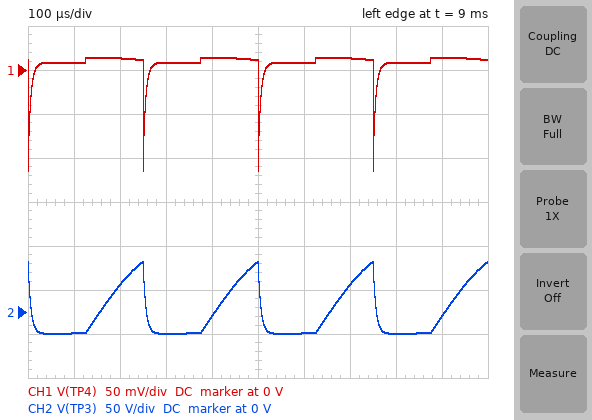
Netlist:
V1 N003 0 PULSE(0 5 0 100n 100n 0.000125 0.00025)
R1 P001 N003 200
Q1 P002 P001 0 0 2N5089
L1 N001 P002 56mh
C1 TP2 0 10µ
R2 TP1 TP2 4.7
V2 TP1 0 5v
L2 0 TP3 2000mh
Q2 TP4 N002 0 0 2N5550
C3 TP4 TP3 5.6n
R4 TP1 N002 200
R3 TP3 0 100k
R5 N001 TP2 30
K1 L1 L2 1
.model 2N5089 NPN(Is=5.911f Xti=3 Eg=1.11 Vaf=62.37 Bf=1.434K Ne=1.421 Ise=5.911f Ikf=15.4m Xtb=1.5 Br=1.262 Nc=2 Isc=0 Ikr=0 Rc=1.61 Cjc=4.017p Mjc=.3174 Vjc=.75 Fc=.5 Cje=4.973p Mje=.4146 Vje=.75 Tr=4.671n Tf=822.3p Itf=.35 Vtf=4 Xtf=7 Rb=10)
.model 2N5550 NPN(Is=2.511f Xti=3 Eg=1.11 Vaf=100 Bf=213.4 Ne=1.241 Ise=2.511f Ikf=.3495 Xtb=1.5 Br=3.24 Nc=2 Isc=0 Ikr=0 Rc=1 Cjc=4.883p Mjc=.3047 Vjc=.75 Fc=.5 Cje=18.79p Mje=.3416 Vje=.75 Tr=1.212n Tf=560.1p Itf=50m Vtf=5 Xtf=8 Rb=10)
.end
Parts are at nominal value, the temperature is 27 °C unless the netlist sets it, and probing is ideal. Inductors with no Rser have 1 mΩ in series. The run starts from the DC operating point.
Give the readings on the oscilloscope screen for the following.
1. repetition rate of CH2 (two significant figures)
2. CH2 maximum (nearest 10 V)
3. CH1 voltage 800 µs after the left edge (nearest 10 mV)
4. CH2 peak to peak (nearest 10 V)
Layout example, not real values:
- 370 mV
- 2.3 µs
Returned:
- 4.0 kHz
- 60 V
- 10 mV
- 80 V
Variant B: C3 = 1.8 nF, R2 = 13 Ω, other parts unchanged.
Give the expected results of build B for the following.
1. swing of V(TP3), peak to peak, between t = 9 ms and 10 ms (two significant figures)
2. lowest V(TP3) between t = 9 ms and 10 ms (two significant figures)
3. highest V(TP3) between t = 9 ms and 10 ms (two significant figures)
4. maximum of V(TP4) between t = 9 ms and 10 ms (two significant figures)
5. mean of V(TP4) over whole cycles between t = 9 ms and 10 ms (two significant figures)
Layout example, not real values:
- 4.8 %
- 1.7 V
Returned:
- 79 V
- -28 V
- 51 V
- 11 mV
- 8.2 mV
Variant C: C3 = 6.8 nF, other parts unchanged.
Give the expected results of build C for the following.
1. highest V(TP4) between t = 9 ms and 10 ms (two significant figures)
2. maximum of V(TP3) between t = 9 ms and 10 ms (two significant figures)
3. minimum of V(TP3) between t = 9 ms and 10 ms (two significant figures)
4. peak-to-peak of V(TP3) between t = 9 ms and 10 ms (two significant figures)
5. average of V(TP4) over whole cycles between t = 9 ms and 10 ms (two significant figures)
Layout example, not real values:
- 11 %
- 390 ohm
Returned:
- 15 mV
- 55 V
- -24 V
- 79 V
- 8.0 mV
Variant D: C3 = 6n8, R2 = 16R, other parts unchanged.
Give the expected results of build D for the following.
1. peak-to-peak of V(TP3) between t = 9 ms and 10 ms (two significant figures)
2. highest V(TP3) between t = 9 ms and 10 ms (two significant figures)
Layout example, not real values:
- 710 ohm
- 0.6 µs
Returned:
- 74 V
- 52 V
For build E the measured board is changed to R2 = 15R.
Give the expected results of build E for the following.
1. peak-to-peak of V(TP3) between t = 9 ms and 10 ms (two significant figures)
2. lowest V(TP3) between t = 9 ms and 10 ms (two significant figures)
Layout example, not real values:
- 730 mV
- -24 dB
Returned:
- 78 V
- -24 V
